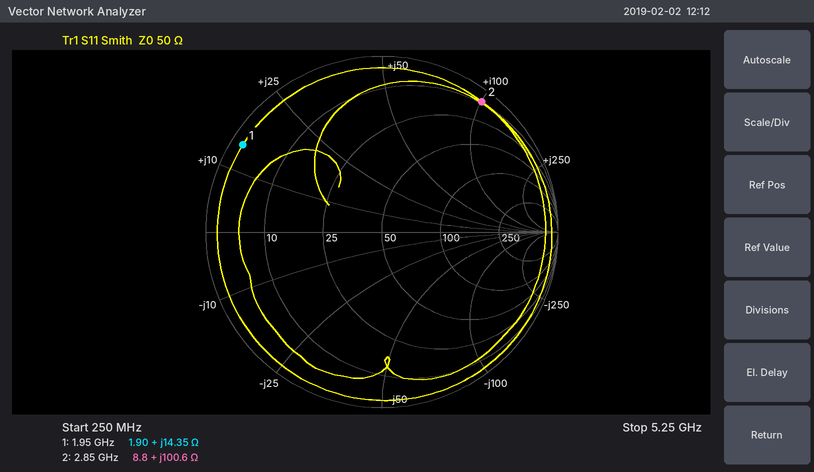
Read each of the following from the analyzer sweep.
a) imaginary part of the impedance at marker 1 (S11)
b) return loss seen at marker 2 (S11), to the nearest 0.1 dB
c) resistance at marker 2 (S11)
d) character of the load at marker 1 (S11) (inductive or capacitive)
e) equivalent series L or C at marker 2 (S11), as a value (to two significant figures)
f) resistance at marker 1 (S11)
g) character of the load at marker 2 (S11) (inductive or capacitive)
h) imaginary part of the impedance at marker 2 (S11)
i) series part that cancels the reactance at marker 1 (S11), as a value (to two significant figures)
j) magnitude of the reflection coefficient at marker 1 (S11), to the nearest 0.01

+14.35 Ω
0.6 dB
8.8 Ω
inductive
5.6 nH
1.90 Ω
inductive
+100.6 Ω
5.7 pF
0.93
